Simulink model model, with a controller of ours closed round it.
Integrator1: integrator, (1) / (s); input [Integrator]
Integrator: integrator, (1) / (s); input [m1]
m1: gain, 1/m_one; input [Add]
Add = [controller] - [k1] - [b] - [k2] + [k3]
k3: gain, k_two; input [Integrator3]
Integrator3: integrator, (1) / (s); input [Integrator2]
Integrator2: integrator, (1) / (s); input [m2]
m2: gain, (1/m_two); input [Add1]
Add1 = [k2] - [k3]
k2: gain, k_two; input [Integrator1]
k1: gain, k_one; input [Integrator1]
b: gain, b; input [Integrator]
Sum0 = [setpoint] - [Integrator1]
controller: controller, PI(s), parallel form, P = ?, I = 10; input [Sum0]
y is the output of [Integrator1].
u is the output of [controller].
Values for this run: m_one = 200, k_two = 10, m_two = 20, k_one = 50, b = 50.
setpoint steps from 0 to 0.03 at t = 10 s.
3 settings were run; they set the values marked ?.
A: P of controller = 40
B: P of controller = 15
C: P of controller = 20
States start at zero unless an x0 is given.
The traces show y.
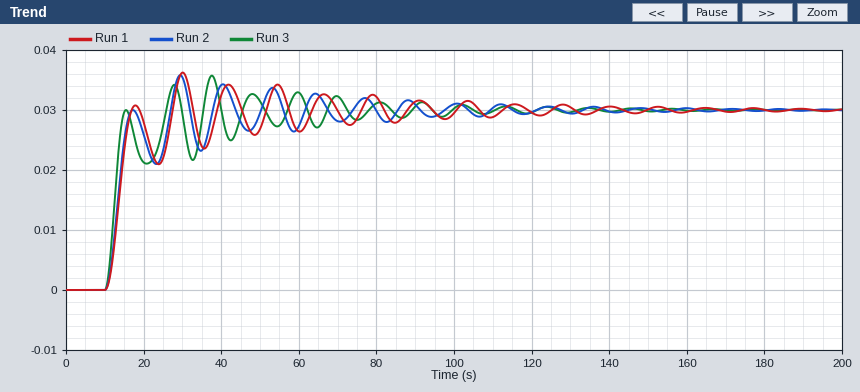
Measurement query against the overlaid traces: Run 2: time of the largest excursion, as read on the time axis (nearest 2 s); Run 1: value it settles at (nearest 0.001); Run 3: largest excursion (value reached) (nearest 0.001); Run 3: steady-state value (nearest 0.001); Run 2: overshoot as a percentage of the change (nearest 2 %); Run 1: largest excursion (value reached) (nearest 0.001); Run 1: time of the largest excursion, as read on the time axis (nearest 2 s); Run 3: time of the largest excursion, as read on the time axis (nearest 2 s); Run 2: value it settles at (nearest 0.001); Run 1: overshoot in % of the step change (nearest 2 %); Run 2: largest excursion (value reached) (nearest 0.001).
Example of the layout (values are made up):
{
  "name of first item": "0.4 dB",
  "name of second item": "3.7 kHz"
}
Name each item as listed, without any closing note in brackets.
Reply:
{
  "Run 2: time of the largest excursion, as read on the time axis": "30 s",
  "Run 1: value it settles at": "0.030",
  "Run 3: largest excursion (value reached)": "0.036",
  "Run 3: steady-state value": "0.030",
  "Run 2: overshoot as a percentage of the change": "20 %",
  "Run 1: largest excursion (value reached)": "0.036",
  "Run 1: time of the largest excursion, as read on the time axis": "30 s",
  "Run 3: time of the largest excursion, as read on the time axis": "38 s",
  "Run 2: value it settles at": "0.030",
  "Run 1: overshoot in % of the step change": "20 %",
  "Run 2: largest excursion (value reached)": "0.036"
}
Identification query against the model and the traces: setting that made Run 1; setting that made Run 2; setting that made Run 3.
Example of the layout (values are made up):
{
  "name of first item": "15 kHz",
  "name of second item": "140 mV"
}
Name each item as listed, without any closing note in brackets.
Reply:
{
  "setting that made Run 1": "B",
  "setting that made Run 2": "C",
  "setting that made Run 3": "A"
}
